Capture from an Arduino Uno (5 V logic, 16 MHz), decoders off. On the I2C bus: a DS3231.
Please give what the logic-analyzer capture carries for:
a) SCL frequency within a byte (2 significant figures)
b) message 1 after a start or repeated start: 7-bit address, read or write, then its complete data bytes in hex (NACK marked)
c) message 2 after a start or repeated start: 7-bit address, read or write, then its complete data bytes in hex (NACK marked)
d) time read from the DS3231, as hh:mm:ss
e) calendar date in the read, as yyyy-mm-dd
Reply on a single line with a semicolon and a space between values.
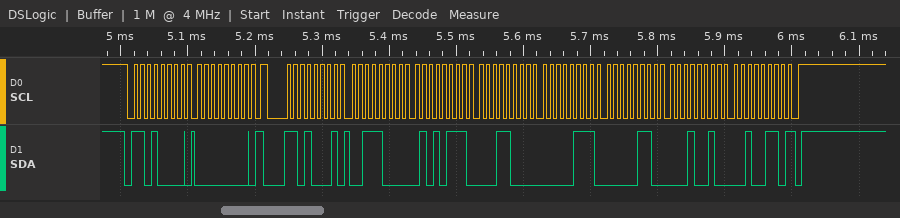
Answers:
100 kHz; 0x68 write: 00; 0x68 read: 38 57 18 07 06 12 26 NACK; 18:57:38; 2026-12-06
